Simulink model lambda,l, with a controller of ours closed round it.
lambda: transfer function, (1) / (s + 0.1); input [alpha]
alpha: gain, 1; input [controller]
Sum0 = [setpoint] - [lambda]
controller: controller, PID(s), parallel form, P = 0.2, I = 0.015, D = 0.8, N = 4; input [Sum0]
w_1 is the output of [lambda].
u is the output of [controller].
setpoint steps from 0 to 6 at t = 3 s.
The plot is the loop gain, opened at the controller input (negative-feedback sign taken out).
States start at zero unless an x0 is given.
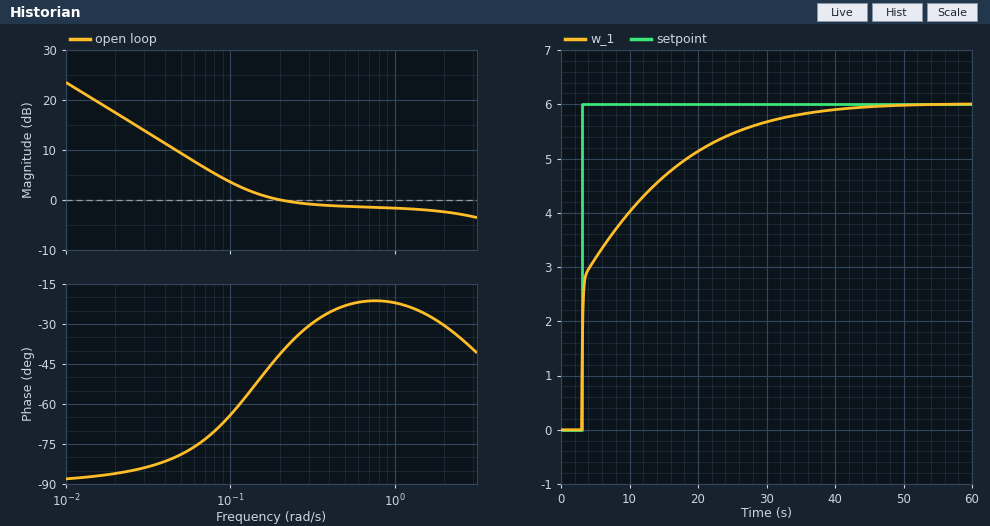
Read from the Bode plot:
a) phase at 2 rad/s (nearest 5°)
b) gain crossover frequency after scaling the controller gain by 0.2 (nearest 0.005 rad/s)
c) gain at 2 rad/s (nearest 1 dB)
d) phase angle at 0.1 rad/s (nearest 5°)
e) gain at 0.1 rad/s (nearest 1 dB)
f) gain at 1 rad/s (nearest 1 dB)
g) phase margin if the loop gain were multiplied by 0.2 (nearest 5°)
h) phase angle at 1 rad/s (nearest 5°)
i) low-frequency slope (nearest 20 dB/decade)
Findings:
-30°
0.030 rad/s
-2 dB
-65°
4 dB
-2 dB
95°
-20°
-20 dB/decade
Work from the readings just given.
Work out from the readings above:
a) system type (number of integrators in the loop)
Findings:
1
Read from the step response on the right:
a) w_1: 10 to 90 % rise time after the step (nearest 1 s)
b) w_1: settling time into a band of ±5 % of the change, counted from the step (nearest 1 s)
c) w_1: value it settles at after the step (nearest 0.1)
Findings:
21 s
28 s
6.0
